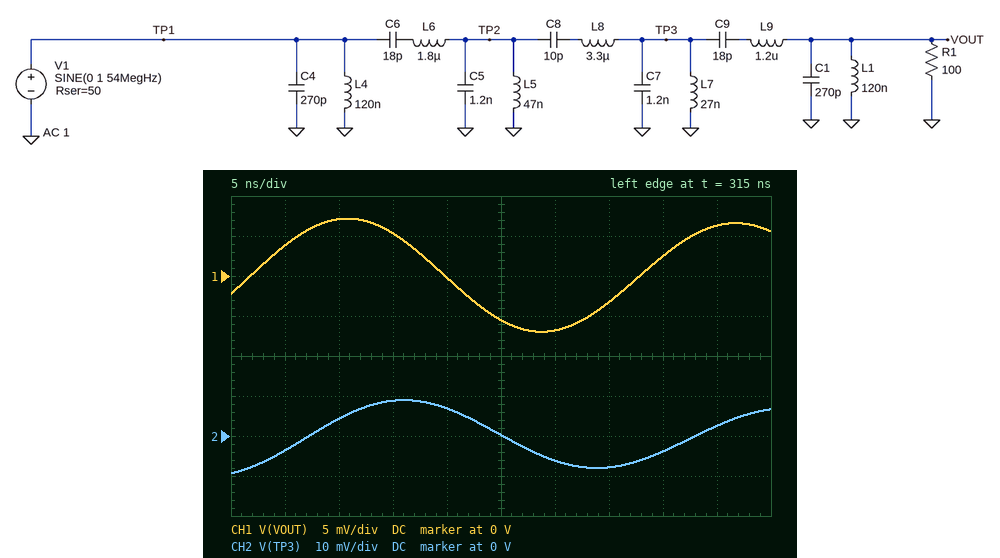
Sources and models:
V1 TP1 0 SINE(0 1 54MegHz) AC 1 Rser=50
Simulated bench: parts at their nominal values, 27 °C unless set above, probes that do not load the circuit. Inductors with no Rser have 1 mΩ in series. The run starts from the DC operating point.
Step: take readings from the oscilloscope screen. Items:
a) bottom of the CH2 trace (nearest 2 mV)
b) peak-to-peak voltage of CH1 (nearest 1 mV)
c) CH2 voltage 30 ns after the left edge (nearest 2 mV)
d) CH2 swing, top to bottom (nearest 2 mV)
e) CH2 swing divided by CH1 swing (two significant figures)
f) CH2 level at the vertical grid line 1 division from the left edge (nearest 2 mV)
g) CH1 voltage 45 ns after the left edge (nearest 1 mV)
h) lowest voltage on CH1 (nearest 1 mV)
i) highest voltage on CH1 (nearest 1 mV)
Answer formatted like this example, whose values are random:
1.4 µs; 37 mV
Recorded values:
-10 mV; 14 mV; -6 mV; 18 mV; 1.3; -4 mV; 6 mV; -7 mV; 7 mV
